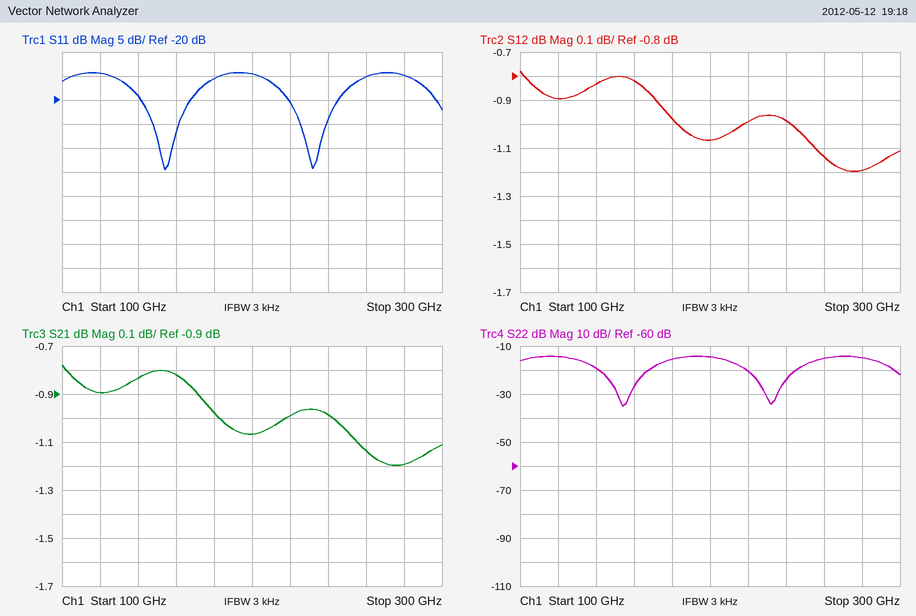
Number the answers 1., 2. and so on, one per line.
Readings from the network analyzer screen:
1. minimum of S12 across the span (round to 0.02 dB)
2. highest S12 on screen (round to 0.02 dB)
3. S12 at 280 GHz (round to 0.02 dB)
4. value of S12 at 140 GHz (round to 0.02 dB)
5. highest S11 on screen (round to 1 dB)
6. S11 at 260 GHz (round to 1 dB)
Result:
1. -1.20 dB
2. -0.78 dB
3. -1.20 dB
4. -0.84 dB
5. -14 dB
6. -15 dB
